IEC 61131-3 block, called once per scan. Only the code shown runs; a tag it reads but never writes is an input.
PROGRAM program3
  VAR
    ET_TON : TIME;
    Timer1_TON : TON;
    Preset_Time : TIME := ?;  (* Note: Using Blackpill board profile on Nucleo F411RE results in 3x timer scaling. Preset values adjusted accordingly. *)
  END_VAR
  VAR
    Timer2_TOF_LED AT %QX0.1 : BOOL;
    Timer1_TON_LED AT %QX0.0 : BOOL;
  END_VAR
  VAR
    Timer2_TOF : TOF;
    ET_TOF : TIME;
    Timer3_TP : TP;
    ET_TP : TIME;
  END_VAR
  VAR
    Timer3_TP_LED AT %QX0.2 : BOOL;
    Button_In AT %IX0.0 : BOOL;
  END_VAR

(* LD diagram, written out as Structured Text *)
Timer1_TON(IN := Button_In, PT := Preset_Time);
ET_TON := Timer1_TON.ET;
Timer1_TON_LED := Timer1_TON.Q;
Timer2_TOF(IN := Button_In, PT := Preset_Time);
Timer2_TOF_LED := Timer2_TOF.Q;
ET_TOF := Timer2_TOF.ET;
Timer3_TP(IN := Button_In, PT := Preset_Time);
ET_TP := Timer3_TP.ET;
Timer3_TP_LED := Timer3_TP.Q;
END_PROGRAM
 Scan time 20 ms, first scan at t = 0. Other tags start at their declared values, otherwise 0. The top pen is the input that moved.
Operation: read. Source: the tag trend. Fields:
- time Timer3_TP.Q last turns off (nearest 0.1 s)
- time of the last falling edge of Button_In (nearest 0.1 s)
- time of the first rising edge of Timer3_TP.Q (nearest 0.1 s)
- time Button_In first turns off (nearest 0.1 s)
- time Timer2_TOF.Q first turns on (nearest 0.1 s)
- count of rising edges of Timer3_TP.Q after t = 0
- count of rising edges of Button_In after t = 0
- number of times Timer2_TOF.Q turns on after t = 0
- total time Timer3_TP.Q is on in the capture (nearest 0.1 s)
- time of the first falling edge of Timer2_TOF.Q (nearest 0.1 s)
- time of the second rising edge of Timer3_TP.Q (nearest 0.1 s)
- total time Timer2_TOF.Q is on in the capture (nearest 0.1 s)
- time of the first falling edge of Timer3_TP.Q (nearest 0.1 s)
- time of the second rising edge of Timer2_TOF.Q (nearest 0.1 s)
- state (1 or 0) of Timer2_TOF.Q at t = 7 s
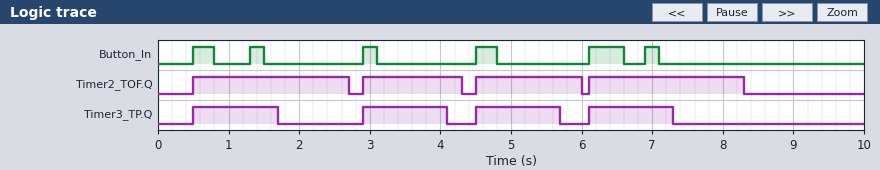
7.3 s
7.1 s
0.5 s
0.8 s
0.5 s
4
6
4
4.8 s
2.7 s
2.9 s
7.3 s
1.7 s
2.9 s
1
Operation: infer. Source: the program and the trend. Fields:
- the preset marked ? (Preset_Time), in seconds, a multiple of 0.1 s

1.2 s
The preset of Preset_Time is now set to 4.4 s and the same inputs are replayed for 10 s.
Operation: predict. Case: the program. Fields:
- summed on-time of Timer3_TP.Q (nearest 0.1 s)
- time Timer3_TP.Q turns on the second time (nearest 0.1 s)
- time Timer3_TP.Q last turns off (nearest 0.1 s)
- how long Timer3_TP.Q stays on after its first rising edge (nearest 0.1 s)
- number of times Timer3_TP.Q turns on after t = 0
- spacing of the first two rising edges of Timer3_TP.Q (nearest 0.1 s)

8.3 s
6.1 s
4.9 s
4.4 s
2
5.6 s
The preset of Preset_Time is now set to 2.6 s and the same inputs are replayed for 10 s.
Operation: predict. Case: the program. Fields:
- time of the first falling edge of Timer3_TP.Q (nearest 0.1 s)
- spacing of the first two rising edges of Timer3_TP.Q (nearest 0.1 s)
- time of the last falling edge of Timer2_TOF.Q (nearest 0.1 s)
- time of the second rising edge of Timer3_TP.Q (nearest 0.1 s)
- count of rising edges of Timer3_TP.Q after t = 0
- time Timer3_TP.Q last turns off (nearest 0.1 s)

3.1 s
4.0 s
9.7 s
4.5 s
2
7.1 s
